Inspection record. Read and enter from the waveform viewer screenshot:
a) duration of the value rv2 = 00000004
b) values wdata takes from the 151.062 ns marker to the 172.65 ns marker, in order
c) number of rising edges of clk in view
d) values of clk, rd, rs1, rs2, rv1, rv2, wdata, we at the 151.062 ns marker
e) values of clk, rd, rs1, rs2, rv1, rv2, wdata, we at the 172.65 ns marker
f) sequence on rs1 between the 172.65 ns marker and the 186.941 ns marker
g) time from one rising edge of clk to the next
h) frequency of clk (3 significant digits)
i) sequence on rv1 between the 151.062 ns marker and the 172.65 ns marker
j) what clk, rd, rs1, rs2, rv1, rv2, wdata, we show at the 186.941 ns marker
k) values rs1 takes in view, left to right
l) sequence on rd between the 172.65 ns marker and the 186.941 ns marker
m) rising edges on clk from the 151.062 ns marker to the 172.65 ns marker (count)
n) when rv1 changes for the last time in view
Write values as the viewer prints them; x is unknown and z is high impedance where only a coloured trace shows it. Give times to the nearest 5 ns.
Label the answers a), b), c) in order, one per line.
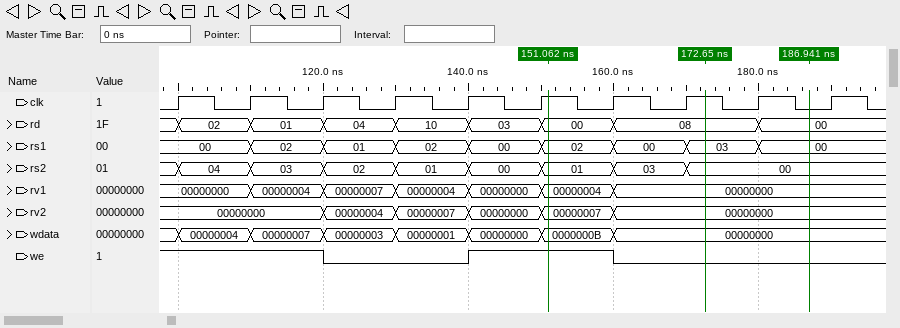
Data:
a) 10 ns
b) 0000000B, 00000000
c) 10
d) clk=1, rd=00, rs1=02, rs2=01, rv1=00000004, rv2=00000007, wdata=0000000B, we=1
e) clk=1, rd=08, rs1=03, rs2=00, rv1=00000000, rv2=00000000, wdata=00000000, we=0
f) 03, 00
g) 10 ns
h) 100 MHz
i) 00000004, 00000000
j) clk=0, rd=00, rs1=00, rs2=00, rv1=00000000, rv2=00000000, wdata=00000000, we=0
k) 00, 02, 01, 02, 00, 02, 00, 03, 00
l) 08, 00
m) 2
n) 160 ns
